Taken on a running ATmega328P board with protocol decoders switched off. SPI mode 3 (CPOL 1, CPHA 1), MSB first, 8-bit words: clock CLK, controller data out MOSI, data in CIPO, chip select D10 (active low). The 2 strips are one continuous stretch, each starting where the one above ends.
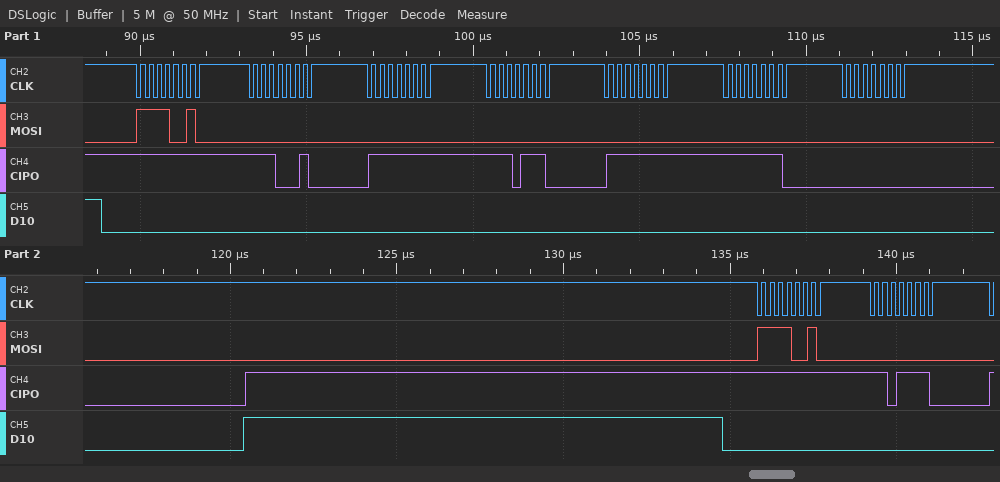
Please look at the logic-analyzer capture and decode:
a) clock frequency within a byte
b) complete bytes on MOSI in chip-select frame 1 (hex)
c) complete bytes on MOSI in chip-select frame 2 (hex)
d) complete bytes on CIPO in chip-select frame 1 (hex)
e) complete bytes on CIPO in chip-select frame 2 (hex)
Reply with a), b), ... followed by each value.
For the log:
a) 4 MHz
b) F2 00 00 00 00 00 00
c) F2 00
d) FF E2 FF EE FF FE 00
e) FF DE
